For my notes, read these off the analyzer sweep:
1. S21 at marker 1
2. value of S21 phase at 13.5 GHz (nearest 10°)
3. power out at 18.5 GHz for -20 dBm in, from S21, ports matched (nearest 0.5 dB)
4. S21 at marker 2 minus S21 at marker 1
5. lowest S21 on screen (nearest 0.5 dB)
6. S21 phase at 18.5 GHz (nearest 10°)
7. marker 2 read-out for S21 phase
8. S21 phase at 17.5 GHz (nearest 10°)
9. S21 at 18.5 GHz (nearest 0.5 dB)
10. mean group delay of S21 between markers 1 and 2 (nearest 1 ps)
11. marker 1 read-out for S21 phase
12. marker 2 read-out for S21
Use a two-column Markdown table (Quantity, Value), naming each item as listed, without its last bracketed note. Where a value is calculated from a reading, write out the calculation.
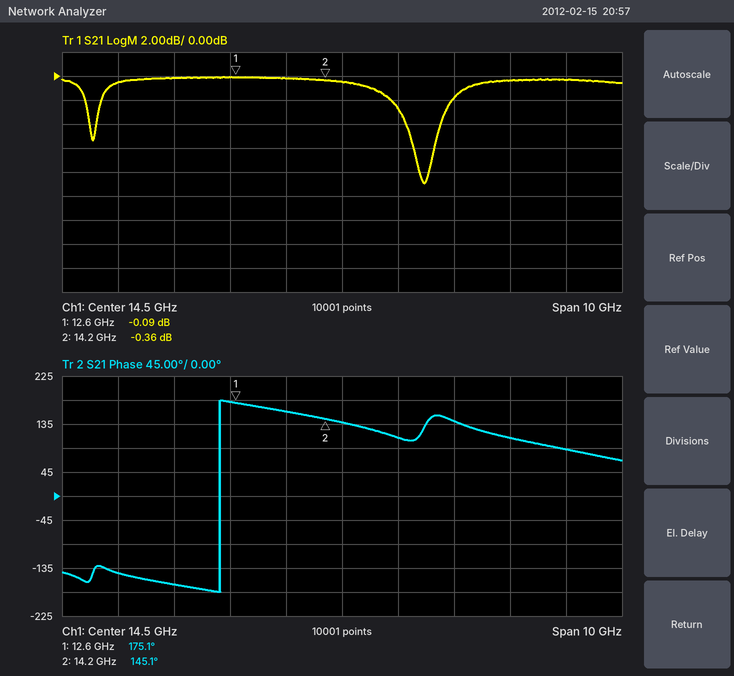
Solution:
| Quantity | Value |
|---|---|
| S21 at marker 1 | -0.09 dB |
| value of S21 phase at 13.5 GHz | 160° |
| power out at 18.5 GHz for -20 dBm in, from S21, ports matched | -20 dBm + (-0.5 dB) = -20.5 dBm |
| S21 at marker 2 minus S21 at marker 1 | -0.36 − (-0.09) = -0.27 dB |
| lowest S21 on screen | -9.0 dB |
| S21 phase at 18.5 GHz | 90° |
| marker 2 read-out for S21 phase | 145.1° |
| S21 phase at 17.5 GHz | 110° |
| S21 at 18.5 GHz | -0.5 dB |
| mean group delay of S21 between markers 1 and 2 | −(145.1° − (175.1°))/(360° × 1.6 GHz) ≈ 52 ps |
| marker 1 read-out for S21 phase | 175.1° |
| marker 2 read-out for S21 | -0.36 dB |
